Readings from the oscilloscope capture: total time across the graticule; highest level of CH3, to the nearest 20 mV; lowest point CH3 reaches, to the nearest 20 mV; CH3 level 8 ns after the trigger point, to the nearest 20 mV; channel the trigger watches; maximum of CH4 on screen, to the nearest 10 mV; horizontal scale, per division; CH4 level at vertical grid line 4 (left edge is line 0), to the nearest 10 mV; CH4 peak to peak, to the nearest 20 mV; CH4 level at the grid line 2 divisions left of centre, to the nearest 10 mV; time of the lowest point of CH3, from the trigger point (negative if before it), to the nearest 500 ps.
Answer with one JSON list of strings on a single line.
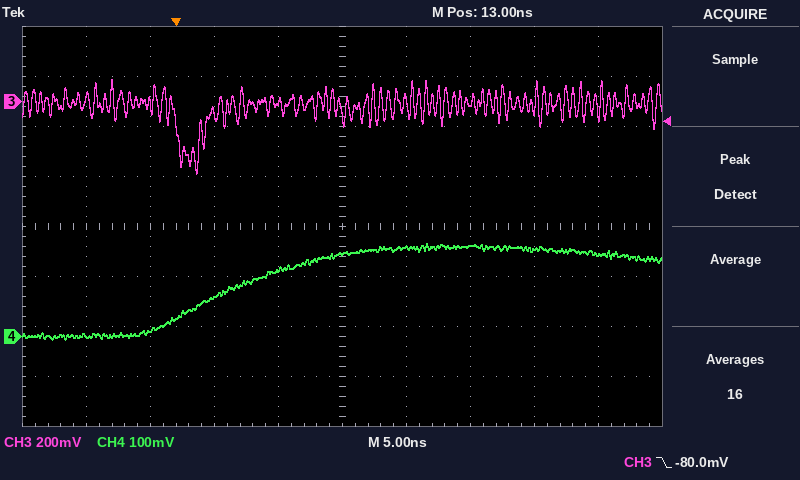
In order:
["50 ns", "80 mV", "-280 mV", "0 mV", "CH3", "190 mV", "5 ns", "130 mV", "200 mV", "80 mV", "+1.5 ns"]
